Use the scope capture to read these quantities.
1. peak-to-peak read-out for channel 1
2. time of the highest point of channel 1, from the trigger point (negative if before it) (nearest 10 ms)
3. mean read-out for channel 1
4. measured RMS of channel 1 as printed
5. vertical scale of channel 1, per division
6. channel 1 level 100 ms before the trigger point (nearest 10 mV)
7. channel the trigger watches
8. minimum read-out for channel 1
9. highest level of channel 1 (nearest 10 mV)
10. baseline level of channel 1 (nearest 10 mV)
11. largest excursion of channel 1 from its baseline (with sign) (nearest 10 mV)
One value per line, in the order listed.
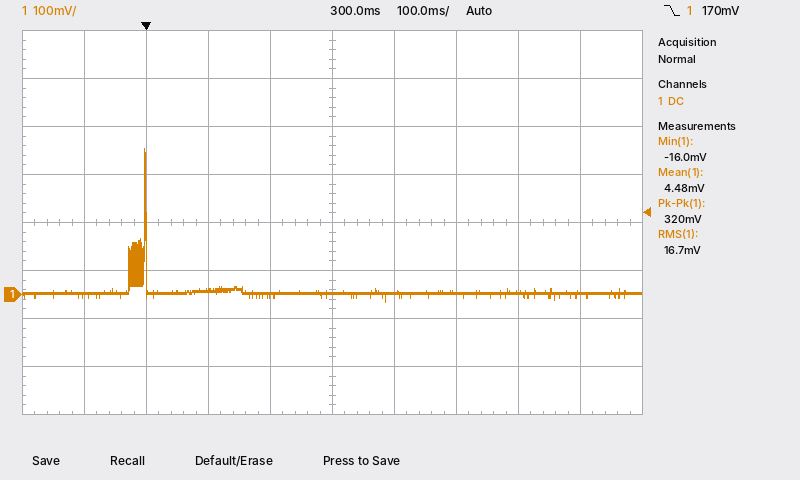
320 mV
0 ms
4.48 mV
16.7 mV
100 mV
0 mV
channel 1
-16.0 mV
300 mV
0 mV
+300 mV
